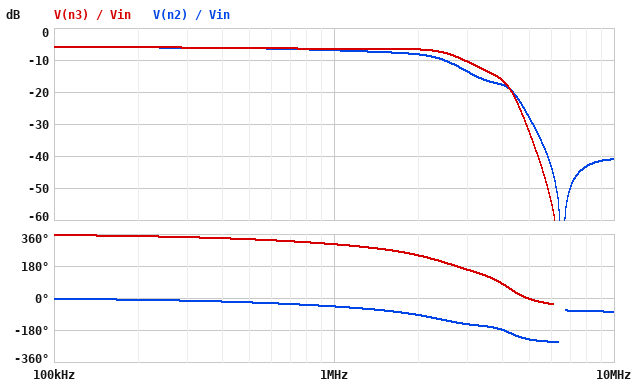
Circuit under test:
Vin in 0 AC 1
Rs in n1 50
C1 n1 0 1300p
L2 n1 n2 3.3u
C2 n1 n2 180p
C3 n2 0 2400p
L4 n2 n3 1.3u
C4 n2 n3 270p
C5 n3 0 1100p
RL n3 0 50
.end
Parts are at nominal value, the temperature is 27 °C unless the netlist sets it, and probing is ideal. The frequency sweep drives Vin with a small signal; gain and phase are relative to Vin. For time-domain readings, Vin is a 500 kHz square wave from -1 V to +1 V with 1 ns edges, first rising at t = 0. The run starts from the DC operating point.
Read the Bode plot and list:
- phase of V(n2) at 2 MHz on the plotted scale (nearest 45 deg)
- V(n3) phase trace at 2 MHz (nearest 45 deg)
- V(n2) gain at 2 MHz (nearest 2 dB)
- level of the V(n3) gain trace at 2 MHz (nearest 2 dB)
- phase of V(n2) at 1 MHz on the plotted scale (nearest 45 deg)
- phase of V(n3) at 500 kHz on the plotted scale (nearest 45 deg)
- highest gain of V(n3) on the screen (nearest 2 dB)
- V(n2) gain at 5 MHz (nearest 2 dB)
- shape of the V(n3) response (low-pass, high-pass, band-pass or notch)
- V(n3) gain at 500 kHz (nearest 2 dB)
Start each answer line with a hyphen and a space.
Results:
- -90 deg
- 225 deg
- -8 dB
- -6 dB
- -45 deg
- 315 deg
- -6 dB
- -28 dB
- low-pass
- -6 dB
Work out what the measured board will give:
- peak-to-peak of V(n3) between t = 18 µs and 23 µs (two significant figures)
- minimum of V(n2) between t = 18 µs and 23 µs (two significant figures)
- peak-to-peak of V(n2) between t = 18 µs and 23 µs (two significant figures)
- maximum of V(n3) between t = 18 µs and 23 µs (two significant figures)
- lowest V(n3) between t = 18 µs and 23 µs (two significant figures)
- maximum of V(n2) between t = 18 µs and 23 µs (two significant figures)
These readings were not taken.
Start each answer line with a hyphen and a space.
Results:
- 1.2 V
- -510 mV
- 1.0 V
- 580 mV
- -580 mV
- 510 mV
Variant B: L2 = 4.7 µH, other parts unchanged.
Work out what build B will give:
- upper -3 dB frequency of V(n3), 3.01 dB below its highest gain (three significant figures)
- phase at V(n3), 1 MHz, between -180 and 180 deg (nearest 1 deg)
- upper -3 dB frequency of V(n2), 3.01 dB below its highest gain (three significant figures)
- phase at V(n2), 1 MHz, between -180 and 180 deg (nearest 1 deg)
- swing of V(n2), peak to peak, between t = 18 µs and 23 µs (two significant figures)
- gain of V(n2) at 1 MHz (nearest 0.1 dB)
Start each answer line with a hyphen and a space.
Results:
- 2.17 MHz
- -65 deg
- 1.91 MHz
- -55 deg
- 1.1 V
- -6.7 dB
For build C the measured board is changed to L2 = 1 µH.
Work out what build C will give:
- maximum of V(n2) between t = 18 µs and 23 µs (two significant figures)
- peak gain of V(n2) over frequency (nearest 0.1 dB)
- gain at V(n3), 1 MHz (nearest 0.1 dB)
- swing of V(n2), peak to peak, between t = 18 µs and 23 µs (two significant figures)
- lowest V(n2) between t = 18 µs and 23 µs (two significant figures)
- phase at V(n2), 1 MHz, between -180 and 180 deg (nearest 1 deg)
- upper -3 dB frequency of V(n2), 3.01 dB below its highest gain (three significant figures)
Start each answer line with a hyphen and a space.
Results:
- 550 mV
- -3.3 dB
- -7.2 dB
- 1.1 V
- -550 mV
- -37 deg
- 5.45 MHz
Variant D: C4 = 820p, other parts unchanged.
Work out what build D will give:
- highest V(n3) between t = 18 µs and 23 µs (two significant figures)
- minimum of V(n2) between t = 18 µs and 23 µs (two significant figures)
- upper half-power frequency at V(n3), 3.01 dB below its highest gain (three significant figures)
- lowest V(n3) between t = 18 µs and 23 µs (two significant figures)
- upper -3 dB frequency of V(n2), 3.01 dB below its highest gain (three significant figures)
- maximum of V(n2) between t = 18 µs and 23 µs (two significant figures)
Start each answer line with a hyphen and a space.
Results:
- 630 mV
- -520 mV
- 3.01 MHz
- -630 mV
- 2.29 MHz
- 520 mV
